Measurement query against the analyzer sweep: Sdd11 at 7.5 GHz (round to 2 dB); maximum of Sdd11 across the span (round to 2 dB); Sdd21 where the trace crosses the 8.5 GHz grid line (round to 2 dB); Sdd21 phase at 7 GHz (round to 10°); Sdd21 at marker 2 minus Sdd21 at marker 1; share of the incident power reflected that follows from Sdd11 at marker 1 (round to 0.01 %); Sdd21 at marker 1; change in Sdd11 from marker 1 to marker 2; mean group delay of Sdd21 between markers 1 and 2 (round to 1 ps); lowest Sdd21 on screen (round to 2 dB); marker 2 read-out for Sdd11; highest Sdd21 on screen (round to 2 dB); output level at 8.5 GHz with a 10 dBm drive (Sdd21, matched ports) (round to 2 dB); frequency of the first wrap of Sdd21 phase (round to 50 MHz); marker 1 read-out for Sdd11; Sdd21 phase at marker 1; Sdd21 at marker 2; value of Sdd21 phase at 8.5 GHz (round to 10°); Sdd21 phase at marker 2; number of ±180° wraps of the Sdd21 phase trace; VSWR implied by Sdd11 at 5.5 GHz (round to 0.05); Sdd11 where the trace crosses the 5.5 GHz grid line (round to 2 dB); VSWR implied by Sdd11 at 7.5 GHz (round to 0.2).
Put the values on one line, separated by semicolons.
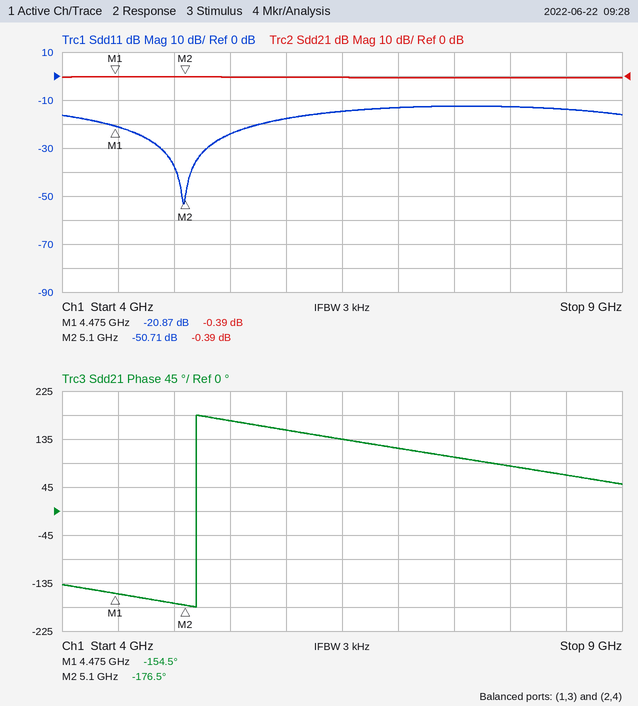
-12 dB; -12 dB; 0 dB; 120°; 0.00 dB; 0.82 %; -0.39 dB; -29.84 dB; 98 ps; 0 dB; -50.71 dB; 0 dB; 10 dBm; 5.20 GHz; -20.87 dB; -154.5°; -0.39 dB; 70°; -176.5°; 1; 1.15; -24 dB; 1.6
